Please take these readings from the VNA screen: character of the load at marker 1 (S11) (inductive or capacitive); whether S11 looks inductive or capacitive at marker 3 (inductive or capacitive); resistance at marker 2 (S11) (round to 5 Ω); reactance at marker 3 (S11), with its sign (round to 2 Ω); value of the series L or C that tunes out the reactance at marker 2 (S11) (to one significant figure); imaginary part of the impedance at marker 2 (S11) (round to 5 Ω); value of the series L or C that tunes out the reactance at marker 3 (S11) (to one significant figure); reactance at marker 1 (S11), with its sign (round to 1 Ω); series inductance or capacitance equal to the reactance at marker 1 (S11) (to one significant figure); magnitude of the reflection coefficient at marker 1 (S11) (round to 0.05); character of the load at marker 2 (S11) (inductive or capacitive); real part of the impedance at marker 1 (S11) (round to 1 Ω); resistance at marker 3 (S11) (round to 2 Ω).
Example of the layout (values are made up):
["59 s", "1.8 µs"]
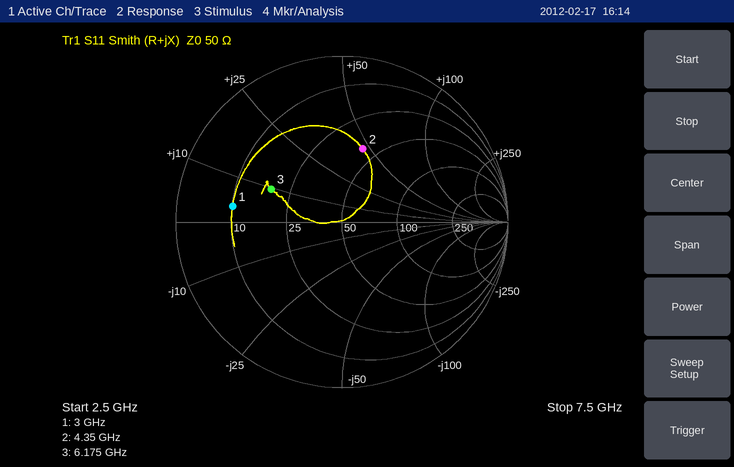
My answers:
["inductive", "inductive", "40 Ω", "+10 Ω", "800 fF", "+45 Ω", "3 pF", "+3 Ω", "200 pH", "0.65", "inductive", "10 Ω", "18 Ω"]
